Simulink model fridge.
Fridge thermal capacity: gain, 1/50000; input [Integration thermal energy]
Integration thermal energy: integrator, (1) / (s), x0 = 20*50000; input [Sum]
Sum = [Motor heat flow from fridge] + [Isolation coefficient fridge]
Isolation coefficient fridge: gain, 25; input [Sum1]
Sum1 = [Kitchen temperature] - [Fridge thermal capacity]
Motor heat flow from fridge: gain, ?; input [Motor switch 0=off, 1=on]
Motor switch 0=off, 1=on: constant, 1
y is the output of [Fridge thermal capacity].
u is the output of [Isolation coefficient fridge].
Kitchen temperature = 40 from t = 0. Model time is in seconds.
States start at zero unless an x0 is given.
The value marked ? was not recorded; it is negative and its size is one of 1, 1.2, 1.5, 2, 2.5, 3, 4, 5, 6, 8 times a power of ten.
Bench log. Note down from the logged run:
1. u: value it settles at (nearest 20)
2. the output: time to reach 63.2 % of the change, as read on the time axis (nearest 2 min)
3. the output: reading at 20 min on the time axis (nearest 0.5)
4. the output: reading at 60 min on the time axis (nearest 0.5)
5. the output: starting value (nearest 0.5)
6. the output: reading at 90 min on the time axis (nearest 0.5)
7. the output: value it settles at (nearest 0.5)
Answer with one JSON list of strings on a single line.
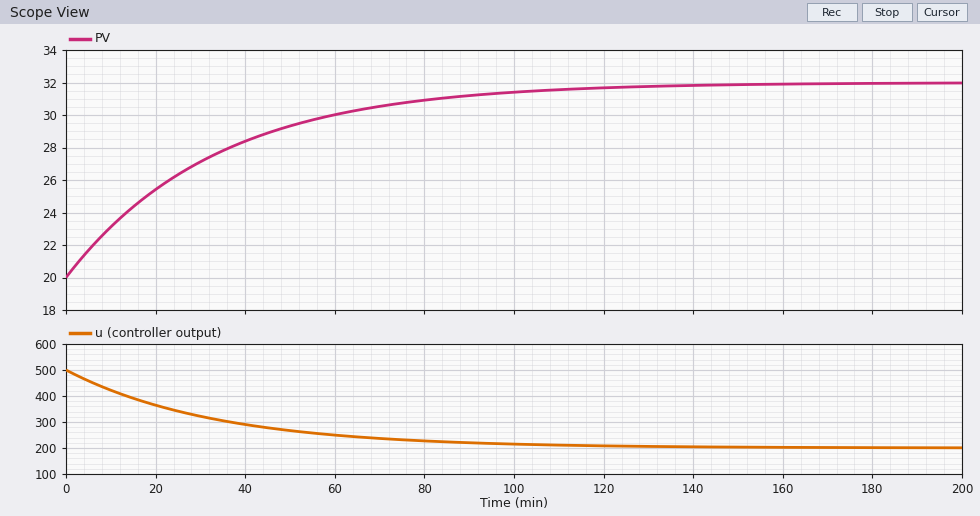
["200", "34 min", "25.5", "30.0", "20.0", "31.0", "32.0"]
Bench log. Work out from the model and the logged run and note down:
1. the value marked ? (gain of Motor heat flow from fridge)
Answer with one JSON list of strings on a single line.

["-200"]
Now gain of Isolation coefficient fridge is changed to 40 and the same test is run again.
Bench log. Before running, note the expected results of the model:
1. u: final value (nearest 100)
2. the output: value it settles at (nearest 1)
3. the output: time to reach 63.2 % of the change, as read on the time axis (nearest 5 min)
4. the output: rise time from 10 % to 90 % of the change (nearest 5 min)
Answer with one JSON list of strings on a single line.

["200", "35", "20 min", "45 min"]
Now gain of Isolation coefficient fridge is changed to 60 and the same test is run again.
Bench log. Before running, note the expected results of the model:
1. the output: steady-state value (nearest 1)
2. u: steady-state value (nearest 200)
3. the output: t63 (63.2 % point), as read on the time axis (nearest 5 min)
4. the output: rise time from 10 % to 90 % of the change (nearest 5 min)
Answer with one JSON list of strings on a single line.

["37", "200", "15 min", "30 min"]
